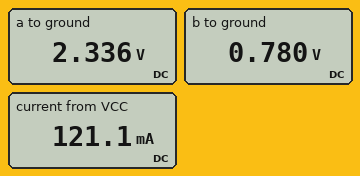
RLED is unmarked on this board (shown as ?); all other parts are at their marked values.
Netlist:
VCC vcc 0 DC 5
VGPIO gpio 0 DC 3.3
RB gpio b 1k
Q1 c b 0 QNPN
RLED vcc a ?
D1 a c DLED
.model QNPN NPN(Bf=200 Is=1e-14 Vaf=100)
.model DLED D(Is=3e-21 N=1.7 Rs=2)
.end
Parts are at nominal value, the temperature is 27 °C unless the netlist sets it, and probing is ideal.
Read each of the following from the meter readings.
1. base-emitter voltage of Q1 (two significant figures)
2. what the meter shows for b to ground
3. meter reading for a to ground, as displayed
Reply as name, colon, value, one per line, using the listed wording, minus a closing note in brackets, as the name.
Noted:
base-emitter voltage of Q1: 780 mV
what the meter shows for b to ground: 0.780 V
meter reading for a to ground, as displayed: 2.336 V
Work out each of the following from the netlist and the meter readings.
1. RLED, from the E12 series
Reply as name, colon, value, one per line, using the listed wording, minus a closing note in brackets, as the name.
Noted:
RLED, from the E12 series: 22 Ω
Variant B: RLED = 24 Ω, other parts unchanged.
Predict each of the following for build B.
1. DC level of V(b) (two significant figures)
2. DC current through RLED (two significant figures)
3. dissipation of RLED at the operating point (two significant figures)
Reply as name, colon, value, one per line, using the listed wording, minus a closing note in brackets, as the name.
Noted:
DC level of V(b): 780 mV
DC current through RLED: 110 mA
dissipation of RLED at the operating point: 300 mW
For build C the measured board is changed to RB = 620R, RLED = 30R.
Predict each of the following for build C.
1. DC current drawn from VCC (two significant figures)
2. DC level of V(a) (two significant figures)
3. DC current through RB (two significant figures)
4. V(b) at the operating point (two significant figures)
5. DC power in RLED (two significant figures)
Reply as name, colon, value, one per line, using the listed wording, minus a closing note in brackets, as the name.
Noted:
DC current drawn from VCC: 92 mA
DC level of V(a): 2.2 V
DC current through RB: 4.1 mA
V(b) at the operating point: 770 mV
DC power in RLED: 250 mW
